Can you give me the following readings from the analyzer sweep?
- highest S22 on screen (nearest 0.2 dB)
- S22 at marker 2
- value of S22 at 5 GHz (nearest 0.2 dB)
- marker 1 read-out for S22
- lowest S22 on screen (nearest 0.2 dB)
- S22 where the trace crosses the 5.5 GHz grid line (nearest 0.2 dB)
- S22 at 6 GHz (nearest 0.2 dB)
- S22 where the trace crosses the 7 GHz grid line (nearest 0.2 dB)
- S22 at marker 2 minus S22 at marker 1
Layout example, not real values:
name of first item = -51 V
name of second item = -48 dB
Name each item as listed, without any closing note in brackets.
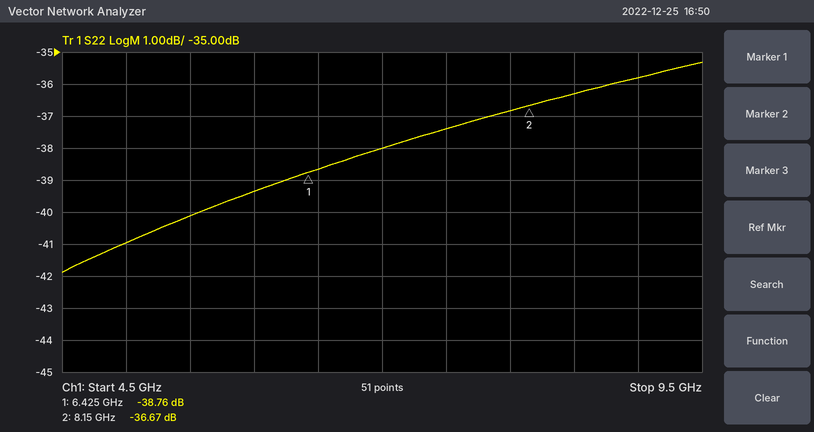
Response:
highest S22 on screen = -35.4 dB
S22 at marker 2 = -36.67 dB
value of S22 at 5 GHz = -41.0 dB
marker 1 read-out for S22 = -38.76 dB
lowest S22 on screen = -41.8 dB
S22 where the trace crosses the 5.5 GHz grid line = -40.2 dB
S22 at 6 GHz = -39.4 dB
S22 where the trace crosses the 7 GHz grid line = -38.0 dB
S22 at marker 2 minus S22 at marker 1 = 2.09 dB
